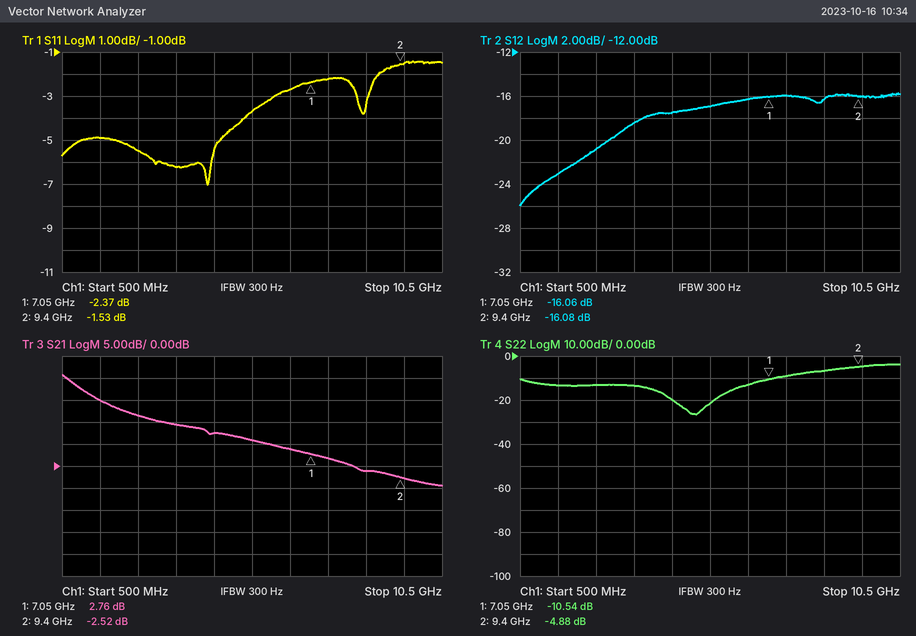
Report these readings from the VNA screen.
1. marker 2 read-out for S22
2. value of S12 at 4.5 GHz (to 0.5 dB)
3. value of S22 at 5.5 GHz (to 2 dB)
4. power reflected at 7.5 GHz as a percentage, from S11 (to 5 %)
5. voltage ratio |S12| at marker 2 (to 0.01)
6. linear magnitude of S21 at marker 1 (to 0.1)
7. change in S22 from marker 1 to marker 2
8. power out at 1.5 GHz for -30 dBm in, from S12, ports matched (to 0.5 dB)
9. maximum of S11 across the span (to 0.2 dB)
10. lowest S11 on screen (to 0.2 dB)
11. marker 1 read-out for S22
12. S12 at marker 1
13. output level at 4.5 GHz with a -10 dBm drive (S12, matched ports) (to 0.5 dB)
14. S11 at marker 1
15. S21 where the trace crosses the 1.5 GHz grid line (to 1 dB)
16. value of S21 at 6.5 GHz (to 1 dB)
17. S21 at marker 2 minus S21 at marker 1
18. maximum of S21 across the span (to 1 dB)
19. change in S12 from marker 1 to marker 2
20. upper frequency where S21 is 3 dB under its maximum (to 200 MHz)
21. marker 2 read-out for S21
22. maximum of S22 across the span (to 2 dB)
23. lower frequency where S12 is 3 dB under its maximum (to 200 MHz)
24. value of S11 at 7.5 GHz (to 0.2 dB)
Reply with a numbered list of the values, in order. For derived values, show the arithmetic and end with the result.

1. -4.88 dB
2. -17.5 dB
3. -22 dB
4. 10^(-2.2/10) ≈ 60 %
5. 10^(-16.08/20) ≈ 0.16
6. 10^(2.76/20) ≈ 1.4
7. -4.88 − (-10.54) = 5.66 dB
8. -30 dBm + (-23.0 dB) = -53.0 dBm
9. -1.4 dB
10. -7.0 dB
11. -10.54 dB
12. -16.06 dB
13. -10 dBm + (-17.5 dB) = -27.5 dBm
14. -2.37 dB
15. 15 dB
16. 4 dB
17. -2.52 − (2.76) = -5.28 dB
18. 21 dB
19. -16.08 − (-16.06) = -0.02 dB
20. 1.0 GHz
21. -2.52 dB
22. -4 dB
23. 3.4 GHz
24. -2.2 dB
